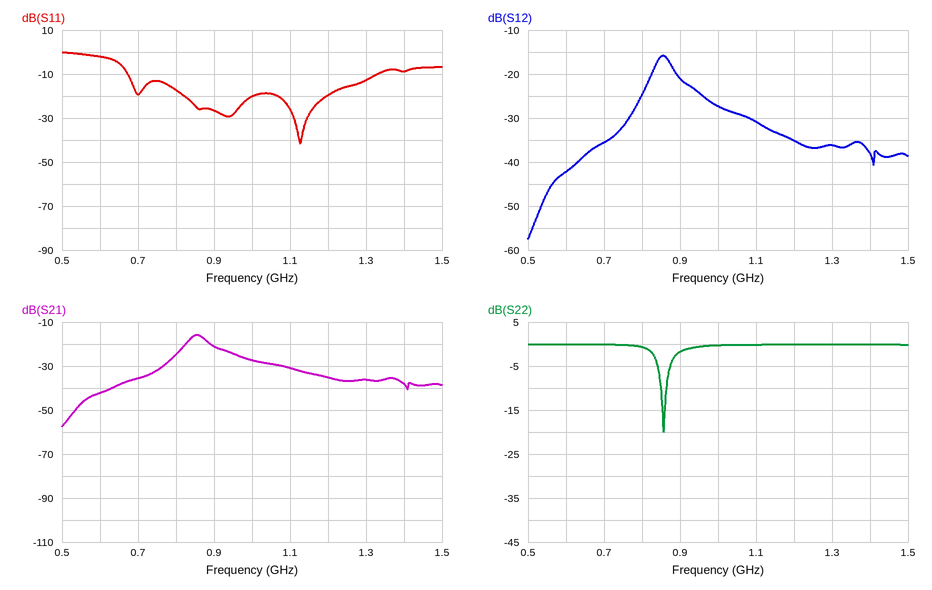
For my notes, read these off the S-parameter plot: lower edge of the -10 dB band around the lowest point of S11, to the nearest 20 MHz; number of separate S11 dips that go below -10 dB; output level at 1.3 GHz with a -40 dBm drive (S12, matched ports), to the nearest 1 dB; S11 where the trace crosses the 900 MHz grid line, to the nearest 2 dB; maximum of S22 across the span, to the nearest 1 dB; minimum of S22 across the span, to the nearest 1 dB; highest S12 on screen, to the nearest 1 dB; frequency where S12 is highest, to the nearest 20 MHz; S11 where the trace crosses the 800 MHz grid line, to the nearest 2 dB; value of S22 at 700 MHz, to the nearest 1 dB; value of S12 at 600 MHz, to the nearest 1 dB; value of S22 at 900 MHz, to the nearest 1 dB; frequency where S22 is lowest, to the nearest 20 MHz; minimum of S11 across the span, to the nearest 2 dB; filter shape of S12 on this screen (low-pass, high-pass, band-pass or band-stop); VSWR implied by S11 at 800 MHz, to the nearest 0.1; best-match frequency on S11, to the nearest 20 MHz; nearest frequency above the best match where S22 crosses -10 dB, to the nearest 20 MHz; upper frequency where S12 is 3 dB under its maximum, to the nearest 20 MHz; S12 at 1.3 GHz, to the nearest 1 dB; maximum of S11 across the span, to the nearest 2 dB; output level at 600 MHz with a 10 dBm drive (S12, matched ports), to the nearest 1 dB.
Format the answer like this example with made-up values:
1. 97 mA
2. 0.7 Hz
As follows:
1. 680 MHz
2. 3
3. -76 dBm
4. -26 dB
5. 0 dB
6. -20 dB
7. -16 dB
8. 860 MHz
9. -18 dB
10. 0 dB
11. -42 dB
12. -2 dB
13. 860 MHz
14. -42 dB
15. band-pass
16. 1.3
17. 1.12 GHz
18. 860 MHz
19. 880 MHz
20. -36 dB
21. 0 dB
22. -32 dBm
